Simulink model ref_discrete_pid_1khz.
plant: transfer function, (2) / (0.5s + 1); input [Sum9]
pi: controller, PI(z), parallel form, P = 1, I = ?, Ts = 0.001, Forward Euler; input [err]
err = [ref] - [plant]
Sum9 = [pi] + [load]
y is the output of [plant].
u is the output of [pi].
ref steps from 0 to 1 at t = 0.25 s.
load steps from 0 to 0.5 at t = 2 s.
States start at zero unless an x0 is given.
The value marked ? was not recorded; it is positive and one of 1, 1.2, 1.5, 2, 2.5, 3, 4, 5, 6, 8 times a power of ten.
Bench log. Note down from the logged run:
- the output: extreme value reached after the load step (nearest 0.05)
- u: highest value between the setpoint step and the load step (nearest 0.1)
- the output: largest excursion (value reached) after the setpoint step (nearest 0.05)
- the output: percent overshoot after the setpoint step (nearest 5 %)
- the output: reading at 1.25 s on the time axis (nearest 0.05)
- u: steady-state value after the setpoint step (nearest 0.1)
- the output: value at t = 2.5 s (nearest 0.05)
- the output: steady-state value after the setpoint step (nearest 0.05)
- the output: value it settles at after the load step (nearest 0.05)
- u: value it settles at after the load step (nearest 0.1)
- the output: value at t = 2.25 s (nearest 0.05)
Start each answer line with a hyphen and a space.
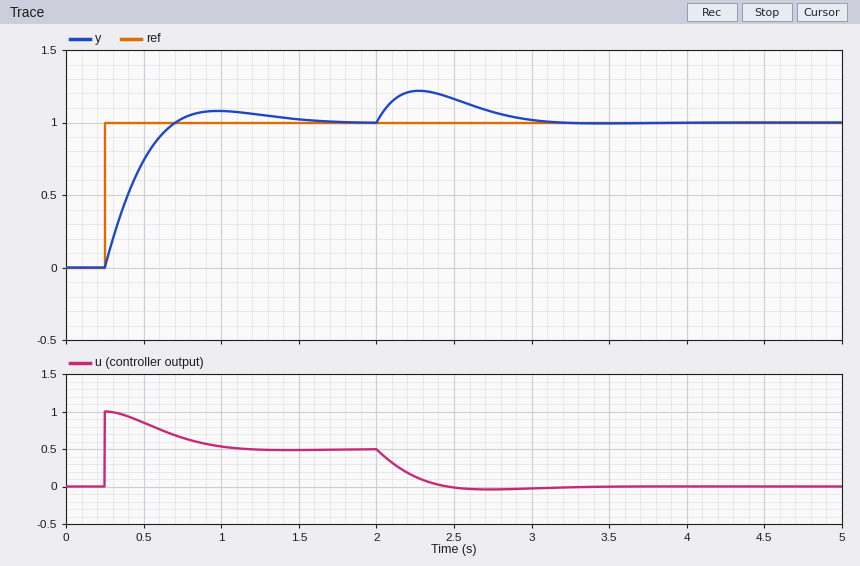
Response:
- 1.20
- 1.0
- 1.10
- 10 %
- 1.05
- 0.5
- 1.15
- 1.00
- 1.00
- 0.0
- 1.20
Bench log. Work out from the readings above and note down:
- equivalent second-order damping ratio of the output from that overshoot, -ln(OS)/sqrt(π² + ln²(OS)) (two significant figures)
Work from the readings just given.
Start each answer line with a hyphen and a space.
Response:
- 0.59
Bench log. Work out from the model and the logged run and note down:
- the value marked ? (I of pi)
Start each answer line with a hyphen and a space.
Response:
- 4
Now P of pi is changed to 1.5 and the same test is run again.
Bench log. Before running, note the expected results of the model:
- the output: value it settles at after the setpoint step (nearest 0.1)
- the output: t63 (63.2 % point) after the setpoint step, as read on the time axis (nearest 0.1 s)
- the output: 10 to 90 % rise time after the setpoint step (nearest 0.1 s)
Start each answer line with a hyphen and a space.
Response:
- 1.0
- 0.4 s
- 0.3 s
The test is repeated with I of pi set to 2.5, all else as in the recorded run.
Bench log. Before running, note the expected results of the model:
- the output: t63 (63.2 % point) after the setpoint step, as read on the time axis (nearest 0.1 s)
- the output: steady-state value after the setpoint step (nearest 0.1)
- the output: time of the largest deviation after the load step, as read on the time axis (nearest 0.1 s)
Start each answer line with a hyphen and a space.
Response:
- 0.5 s
- 1.0
- 2.3 s
